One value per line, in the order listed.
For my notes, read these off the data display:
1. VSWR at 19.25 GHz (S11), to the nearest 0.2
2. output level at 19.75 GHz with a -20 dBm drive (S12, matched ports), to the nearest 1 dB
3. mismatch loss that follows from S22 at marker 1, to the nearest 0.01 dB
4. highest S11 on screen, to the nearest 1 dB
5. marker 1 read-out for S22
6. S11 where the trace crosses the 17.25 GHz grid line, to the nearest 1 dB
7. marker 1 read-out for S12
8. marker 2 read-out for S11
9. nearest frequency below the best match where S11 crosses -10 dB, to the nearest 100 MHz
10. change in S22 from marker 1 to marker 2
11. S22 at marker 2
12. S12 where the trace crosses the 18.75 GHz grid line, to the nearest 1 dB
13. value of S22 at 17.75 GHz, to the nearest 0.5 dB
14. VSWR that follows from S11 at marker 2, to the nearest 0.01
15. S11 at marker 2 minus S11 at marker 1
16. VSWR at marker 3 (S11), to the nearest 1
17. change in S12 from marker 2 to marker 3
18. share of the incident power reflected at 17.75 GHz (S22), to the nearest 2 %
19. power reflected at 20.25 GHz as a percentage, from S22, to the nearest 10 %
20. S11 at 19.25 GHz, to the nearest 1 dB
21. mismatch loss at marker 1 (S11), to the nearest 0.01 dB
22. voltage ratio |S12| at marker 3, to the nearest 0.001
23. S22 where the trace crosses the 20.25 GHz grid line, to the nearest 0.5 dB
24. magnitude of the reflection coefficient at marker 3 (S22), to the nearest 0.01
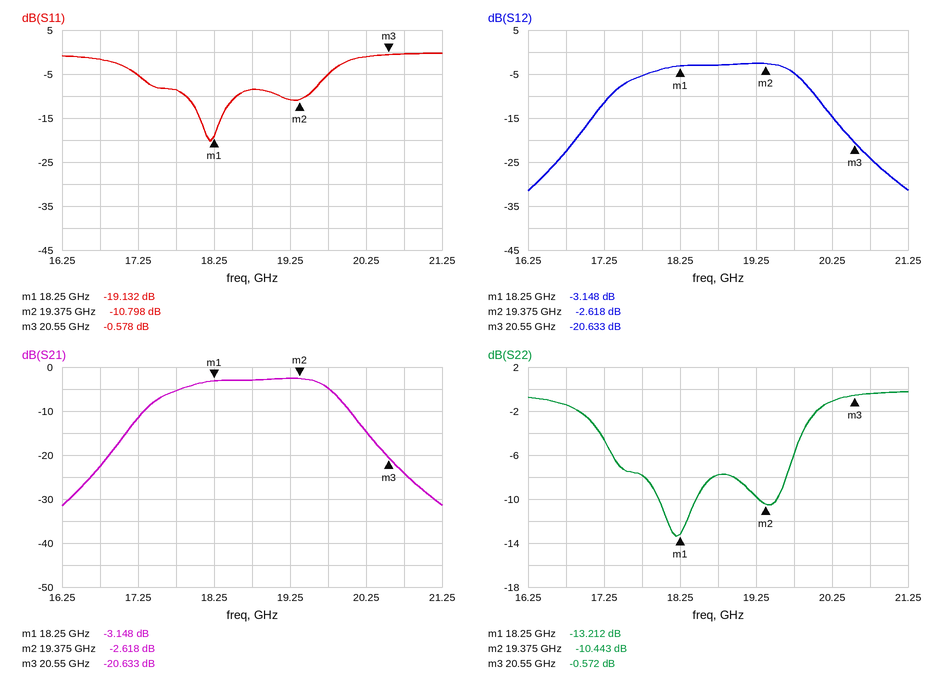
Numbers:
1.8
-25 dBm
0.21 dB
0 dB
-13.212 dB
-5 dB
-3.148 dB
-10.798 dB
17.9 GHz
2.769 dB
-10.443 dB
-3 dB
-8.0 dB
1.81
8.334 dB
30
-18.015 dB
16 %
80 %
-11 dB
0.05 dB
0.093
-1.0 dB
0.94
